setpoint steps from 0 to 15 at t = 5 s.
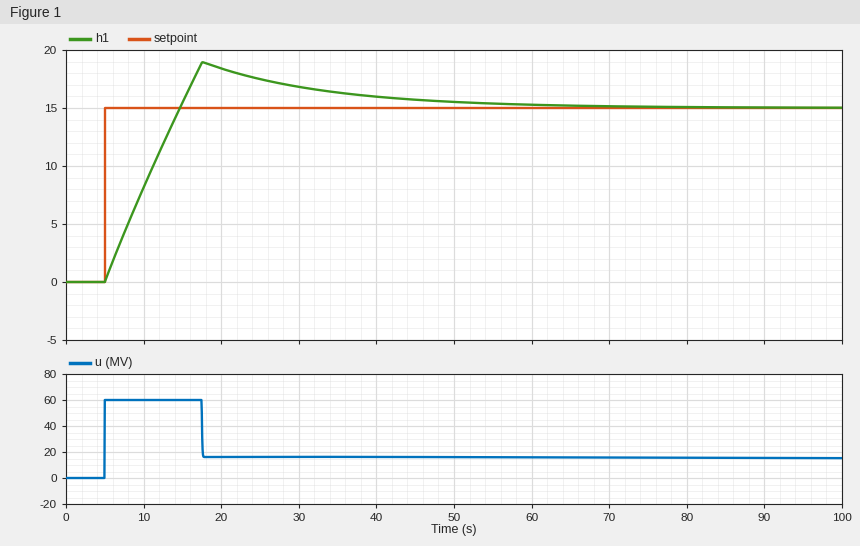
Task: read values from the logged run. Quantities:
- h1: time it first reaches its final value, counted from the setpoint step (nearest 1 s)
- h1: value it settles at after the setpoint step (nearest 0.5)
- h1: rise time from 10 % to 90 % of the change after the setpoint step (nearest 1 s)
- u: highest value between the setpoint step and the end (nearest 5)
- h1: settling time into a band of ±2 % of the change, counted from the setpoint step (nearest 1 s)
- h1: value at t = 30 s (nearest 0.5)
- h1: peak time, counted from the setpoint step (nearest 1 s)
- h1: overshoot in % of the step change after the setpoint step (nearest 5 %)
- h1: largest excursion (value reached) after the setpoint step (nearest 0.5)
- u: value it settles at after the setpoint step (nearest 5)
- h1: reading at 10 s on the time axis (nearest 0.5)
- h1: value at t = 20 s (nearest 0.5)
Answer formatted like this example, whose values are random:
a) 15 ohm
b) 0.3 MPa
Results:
a) 10 s
b) 15.0
c) 8 s
d) 60
e) 54 s
f) 17.0
g) 13 s
h) 25 %
i) 19.0
j) 15
k) 8.0
l) 18.5
